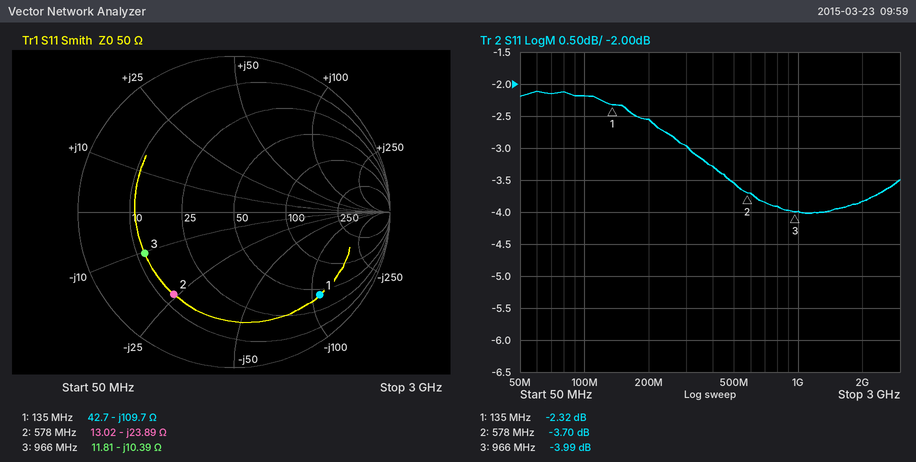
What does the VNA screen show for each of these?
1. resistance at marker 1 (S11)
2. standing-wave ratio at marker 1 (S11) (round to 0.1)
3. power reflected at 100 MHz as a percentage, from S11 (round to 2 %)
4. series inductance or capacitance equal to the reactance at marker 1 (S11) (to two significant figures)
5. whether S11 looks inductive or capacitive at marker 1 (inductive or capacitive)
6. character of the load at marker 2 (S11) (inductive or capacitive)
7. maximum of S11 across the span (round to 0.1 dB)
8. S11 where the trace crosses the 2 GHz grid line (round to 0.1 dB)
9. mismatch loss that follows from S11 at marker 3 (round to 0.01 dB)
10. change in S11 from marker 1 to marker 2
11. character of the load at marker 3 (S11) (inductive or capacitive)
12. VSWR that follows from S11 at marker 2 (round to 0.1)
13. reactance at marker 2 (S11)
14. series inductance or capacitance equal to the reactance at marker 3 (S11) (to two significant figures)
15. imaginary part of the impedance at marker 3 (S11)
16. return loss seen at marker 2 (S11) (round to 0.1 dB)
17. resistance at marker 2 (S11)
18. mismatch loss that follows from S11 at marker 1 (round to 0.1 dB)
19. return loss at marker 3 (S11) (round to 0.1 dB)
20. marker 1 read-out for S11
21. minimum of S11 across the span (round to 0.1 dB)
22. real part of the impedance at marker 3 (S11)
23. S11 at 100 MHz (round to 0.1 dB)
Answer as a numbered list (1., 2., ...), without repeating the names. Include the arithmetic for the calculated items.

1. 42.7 Ω
2. 7.5
3. 10^(-2.2/10) ≈ 60 %
4. C = 1/(2π × 135 MHz × 109.7 Ω) ≈ 11 pF
5. capacitive
6. capacitive
7. -2.1 dB
8. -3.8 dB
9. −10 log10(1 − 10^(-3.99/10)) ≈ 2.21 dB
10. -3.7 − (-2.32) = -1.38 dB
11. capacitive
12. (1 + 0.6531)/(1 − 0.6531) ≈ 4.8
13. -23.89 Ω
14. C = 1/(2π × 966 MHz × 10.39 Ω) ≈ 16 pF
15. -10.39 Ω
16. 3.7 dB
17. 13.02 Ω
18. −10 log10(1 − 10^(-2.32/10)) ≈ 3.8 dB
19. 4.0 dB
20. -2.32 dB
21. -4.0 dB
22. 11.81 Ω
23. -2.2 dB
